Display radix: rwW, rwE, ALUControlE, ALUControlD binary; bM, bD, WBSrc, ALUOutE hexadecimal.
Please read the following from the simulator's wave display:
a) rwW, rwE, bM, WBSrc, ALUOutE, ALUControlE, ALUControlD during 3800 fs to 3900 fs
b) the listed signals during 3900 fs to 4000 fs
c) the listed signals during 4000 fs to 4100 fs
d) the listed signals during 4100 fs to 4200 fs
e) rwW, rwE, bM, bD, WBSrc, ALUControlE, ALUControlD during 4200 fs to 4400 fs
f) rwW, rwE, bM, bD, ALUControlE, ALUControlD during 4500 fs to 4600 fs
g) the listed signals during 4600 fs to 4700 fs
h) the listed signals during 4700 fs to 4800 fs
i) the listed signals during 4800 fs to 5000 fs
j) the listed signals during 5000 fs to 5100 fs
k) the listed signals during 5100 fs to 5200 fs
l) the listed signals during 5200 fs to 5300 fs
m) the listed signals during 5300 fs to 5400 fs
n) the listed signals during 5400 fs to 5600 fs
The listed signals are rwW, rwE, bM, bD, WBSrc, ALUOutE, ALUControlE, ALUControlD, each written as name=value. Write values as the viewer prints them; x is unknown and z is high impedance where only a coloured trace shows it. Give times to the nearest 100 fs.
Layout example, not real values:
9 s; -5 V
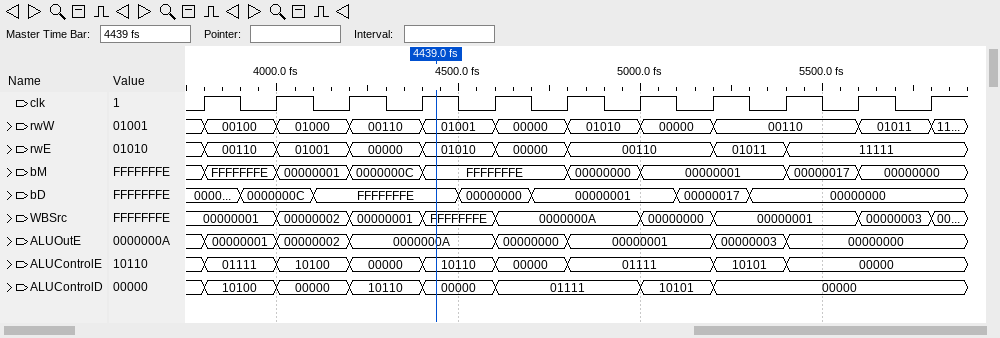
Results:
rwW=00100, rwE=00110, bM=FFFFFFFE, WBSrc=00000001, ALUOutE=00000001, ALUControlE=01111, ALUControlD=10100; rwW=00100, rwE=00110, bM=FFFFFFFE, bD=0000000C, WBSrc=00000001, ALUOutE=00000001, ALUControlE=01111, ALUControlD=10100; rwW=01000, rwE=01001, bM=00000001, bD=0000000C, WBSrc=00000002, ALUOutE=00000002, ALUControlE=10100, ALUControlD=00000; rwW=01000, rwE=01001, bM=00000001, bD=FFFFFFFE, WBSrc=00000002, ALUOutE=00000002, ALUControlE=10100, ALUControlD=00000; rwW=00110, rwE=00000, bM=0000000C, bD=FFFFFFFE, WBSrc=00000001, ALUControlE=00000, ALUControlD=10110; rwW=01001, rwE=01010, bM=FFFFFFFE, bD=00000000, ALUControlE=10110, ALUControlD=00000; rwW=00000, rwE=00000, bM=FFFFFFFE, bD=00000000, WBSrc=0000000A, ALUOutE=00000000, ALUControlE=00000, ALUControlD=01111; rwW=00000, rwE=00000, bM=FFFFFFFE, bD=00000001, WBSrc=0000000A, ALUOutE=00000000, ALUControlE=00000, ALUControlD=01111; rwW=01010, rwE=00110, bM=00000000, bD=00000001, WBSrc=0000000A, ALUOutE=00000001, ALUControlE=01111, ALUControlD=01111; rwW=00000, rwE=00110, bM=00000001, bD=00000001, WBSrc=00000000, ALUOutE=00000001, ALUControlE=01111, ALUControlD=10101; rwW=00000, rwE=00110, bM=00000001, bD=00000017, WBSrc=00000000, ALUOutE=00000001, ALUControlE=01111, ALUControlD=10101; rwW=00110, rwE=01011, bM=00000001, bD=00000017, WBSrc=00000001, ALUOutE=00000003, ALUControlE=10101, ALUControlD=00000; rwW=00110, rwE=01011, bM=00000001, bD=00000000, WBSrc=00000001, ALUOutE=00000003, ALUControlE=10101, ALUControlD=00000; rwW=00110, rwE=11111, bM=00000017, bD=00000000, WBSrc=00000001, ALUOutE=00000000, ALUControlE=00000, ALUControlD=00000
